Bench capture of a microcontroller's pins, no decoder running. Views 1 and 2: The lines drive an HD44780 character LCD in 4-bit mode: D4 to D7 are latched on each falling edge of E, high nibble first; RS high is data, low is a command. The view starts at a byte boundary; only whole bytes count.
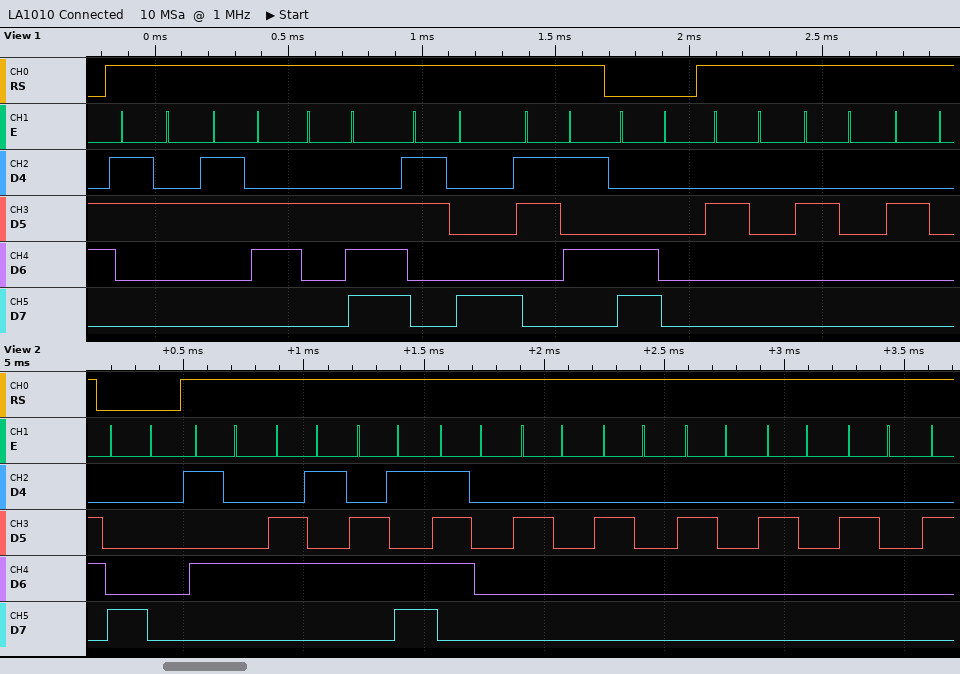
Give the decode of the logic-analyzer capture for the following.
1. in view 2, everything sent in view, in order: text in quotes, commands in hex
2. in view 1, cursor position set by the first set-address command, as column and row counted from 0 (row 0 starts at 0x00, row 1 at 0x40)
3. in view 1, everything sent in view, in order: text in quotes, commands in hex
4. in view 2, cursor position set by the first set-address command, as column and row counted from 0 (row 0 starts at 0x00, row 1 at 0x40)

0x80 "Temp     "
column 0, row 1
"26.85" 0xC0 "   "
column 0, row 0
